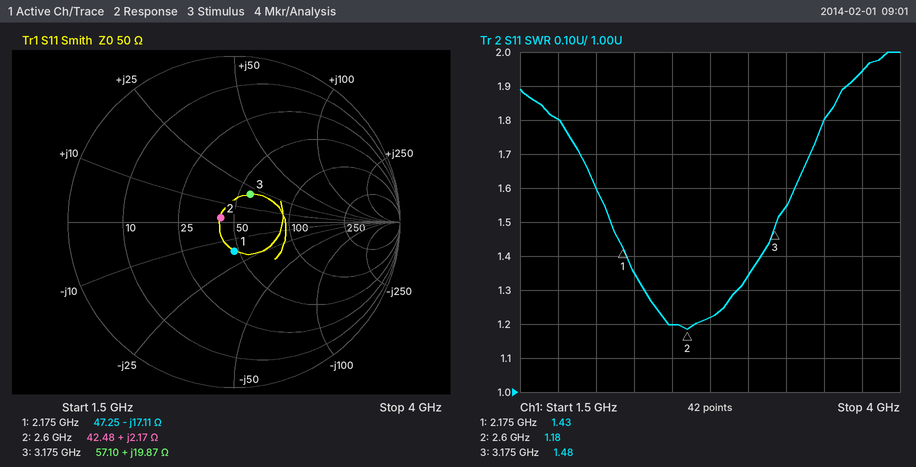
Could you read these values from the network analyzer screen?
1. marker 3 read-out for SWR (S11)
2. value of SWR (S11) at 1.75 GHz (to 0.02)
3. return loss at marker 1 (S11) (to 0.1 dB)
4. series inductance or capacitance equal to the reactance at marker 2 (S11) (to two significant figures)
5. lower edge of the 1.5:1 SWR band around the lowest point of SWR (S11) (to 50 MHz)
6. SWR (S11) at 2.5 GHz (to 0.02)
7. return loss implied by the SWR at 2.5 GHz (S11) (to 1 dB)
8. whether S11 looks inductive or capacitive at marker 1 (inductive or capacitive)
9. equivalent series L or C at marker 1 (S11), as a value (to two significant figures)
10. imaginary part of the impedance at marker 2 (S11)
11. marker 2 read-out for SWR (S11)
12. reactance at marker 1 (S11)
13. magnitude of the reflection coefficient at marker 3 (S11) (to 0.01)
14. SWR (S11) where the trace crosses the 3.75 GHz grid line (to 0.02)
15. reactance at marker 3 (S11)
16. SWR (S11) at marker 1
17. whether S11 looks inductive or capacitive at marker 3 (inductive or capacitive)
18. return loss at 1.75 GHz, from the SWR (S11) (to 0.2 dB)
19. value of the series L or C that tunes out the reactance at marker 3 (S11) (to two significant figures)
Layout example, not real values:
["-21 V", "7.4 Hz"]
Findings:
["1.48", "1.80", "15.1 dB", "130 pH", "2.10 GHz", "1.20", "21 dB", "capacitive", "4.3 pF", "+2.17 Ω", "1.18", "-17.11 Ω", "0.19", "1.94", "+19.87 Ω", "1.43", "inductive", "10.8 dB", "2.5 pF"]
